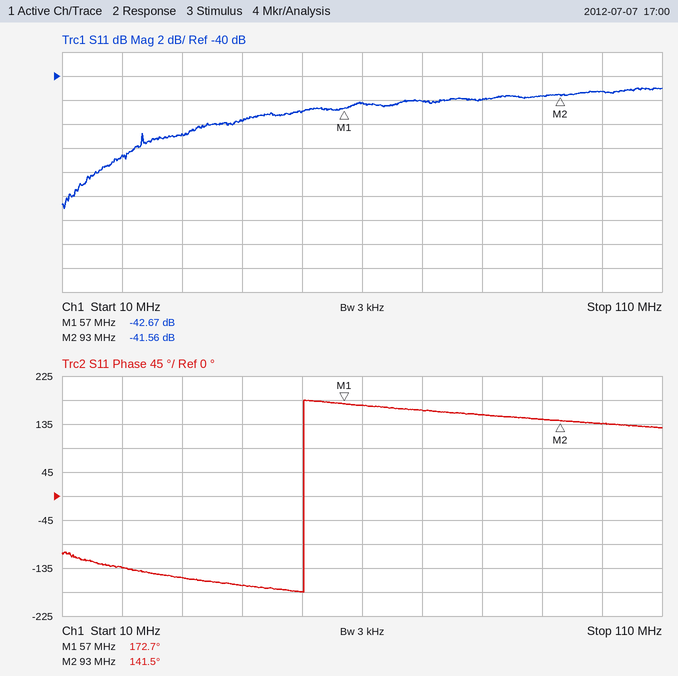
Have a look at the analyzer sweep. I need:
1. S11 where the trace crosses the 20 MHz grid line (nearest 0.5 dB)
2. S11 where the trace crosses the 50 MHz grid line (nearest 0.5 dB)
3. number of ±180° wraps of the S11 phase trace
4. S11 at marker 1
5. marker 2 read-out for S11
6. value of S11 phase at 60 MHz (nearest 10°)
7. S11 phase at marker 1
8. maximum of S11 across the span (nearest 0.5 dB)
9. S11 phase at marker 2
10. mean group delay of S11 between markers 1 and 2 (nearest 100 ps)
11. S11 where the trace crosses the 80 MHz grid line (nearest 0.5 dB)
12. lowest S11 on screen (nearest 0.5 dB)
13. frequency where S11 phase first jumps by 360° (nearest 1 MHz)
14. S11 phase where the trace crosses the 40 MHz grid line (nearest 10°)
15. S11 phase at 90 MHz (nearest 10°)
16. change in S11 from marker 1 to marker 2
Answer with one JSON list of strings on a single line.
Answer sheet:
["-46.5 dB", "-43.0 dB", "1", "-42.67 dB", "-41.56 dB", "170°", "172.7°", "-41.0 dB", "141.5°", "2.4 ns", "-42.0 dB", "-51.0 dB", "50 MHz", "-170°", "140°", "1.11 dB"]
